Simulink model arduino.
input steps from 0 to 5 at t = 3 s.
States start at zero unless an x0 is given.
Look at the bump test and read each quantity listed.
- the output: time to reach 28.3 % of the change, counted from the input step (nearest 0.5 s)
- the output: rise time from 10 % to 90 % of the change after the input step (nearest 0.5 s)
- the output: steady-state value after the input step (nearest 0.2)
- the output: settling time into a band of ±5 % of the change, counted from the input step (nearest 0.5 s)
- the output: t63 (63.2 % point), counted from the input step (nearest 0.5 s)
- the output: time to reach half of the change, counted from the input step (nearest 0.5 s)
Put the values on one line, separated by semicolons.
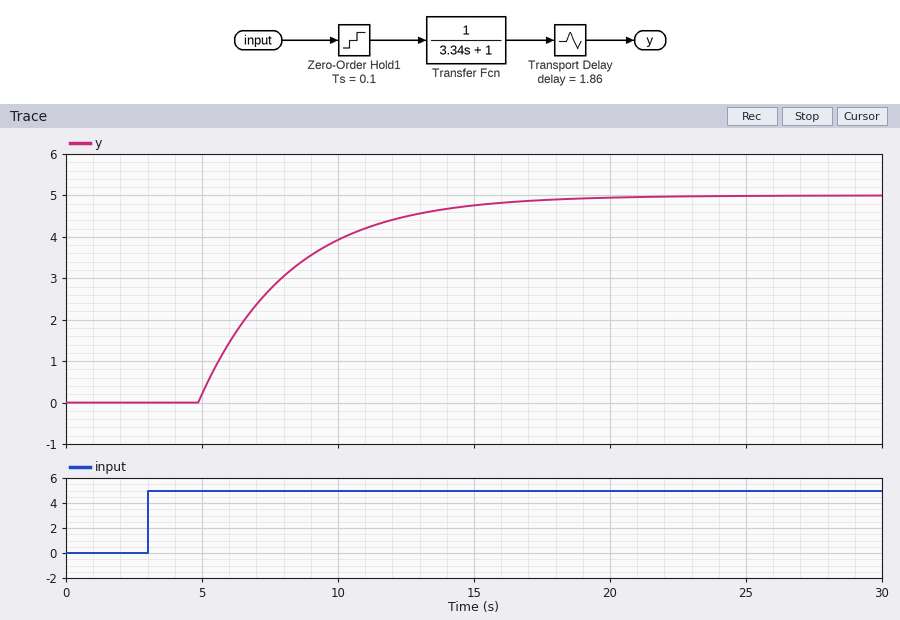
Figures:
3.0 s; 7.5 s; 5.0; 12.0 s; 5.0 s; 4.0 s
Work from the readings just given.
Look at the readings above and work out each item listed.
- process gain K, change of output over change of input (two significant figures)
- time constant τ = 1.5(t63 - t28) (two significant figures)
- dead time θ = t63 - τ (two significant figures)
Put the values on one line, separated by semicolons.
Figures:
1.0; 3.0 s; 2.0 s
